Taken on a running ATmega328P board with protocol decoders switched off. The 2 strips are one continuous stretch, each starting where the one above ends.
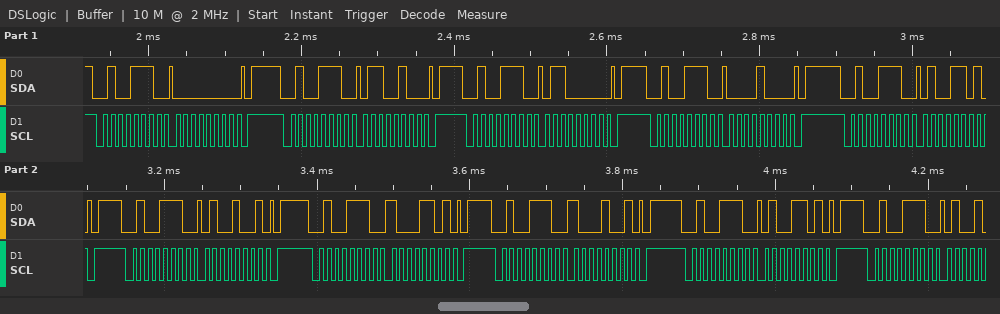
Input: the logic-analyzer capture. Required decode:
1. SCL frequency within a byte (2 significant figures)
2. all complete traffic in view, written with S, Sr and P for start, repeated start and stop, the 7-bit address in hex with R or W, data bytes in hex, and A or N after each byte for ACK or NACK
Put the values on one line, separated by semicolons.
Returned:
100 kHz; S 27W A 00 A P S 27W A 64 A P S 27W A 60 A P S 27W A 08 A P S 27W A 4D A P S 27W A 49 A P S 27W A 8D A P S 27W A 89 A P S 27W A 4D A P S 27W A
